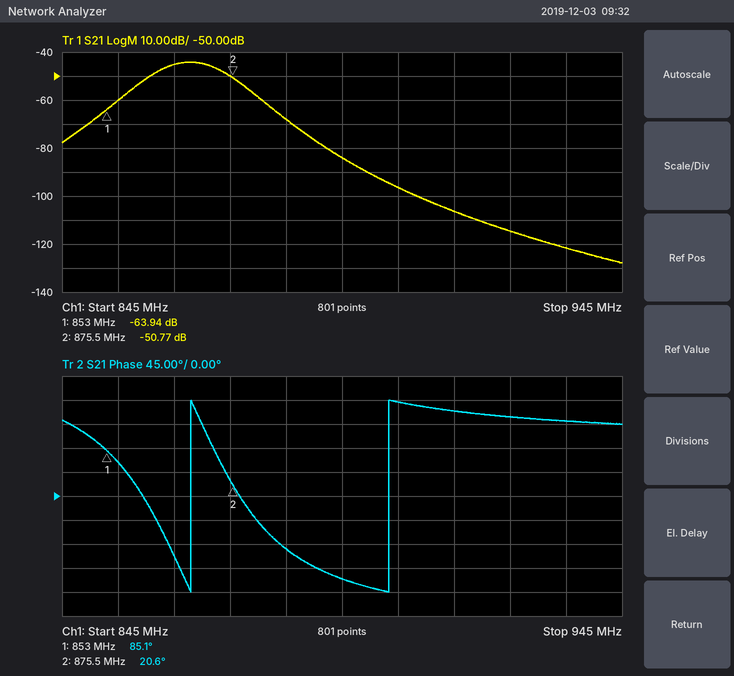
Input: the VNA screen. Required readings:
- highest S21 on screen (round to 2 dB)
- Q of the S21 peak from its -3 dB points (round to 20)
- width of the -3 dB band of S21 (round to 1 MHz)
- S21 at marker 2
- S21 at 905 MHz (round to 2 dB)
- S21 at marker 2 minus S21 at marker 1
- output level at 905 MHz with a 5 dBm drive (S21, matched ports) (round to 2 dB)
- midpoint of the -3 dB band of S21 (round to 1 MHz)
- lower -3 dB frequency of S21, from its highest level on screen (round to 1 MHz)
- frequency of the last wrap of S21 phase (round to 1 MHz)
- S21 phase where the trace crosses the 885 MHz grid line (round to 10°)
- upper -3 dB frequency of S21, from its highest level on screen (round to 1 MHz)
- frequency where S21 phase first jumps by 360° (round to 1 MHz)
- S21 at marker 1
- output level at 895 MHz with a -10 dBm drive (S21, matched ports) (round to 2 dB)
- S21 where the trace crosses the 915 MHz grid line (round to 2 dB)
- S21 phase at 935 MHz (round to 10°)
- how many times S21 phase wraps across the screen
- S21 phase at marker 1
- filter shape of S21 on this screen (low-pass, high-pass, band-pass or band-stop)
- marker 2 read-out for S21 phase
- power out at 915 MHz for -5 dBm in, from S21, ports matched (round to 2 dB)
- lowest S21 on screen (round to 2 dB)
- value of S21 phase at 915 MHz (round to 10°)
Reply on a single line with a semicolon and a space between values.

-44 dB; 80; 10 MHz; -50.77 dB; -96 dB; 13.17 dB; -92 dBm; 868 MHz; 863 MHz; 903 MHz; -100°; 873 MHz; 868 MHz; -63.94 dB; -94 dBm; -106 dB; 140°; 2; 85.1°; band-pass; 20.6°; -112 dBm; -128 dB; 160°
